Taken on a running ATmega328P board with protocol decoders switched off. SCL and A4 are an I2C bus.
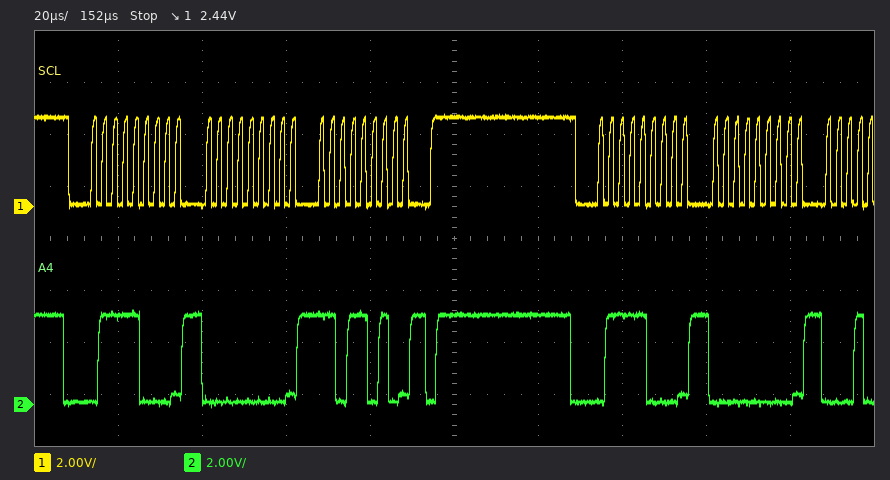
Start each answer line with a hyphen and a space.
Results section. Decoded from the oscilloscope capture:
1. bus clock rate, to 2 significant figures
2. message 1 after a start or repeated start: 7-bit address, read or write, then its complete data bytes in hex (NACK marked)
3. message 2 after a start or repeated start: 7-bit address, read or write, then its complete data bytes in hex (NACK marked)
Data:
- 400 kHz
- 0x3C write: 00 DA
- 0x3C write: 00
